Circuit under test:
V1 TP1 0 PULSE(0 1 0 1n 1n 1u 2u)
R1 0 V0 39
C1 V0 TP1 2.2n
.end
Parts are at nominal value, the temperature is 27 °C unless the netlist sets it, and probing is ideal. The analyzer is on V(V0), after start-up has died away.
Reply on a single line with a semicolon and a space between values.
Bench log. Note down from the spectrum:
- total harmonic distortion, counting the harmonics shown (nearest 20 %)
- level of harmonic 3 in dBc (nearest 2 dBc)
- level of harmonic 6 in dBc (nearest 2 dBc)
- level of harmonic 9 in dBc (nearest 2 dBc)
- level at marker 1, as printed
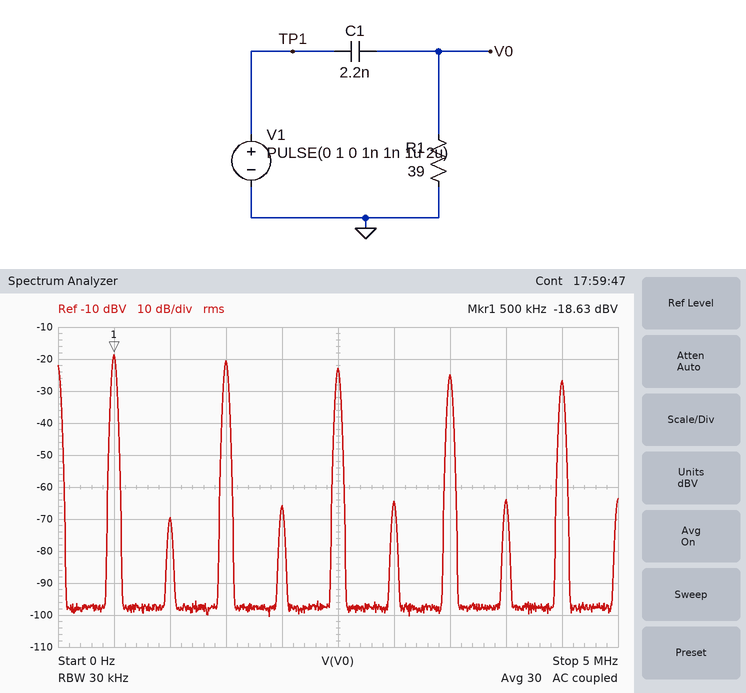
120 %; -2 dBc; -46 dBc; -8 dBc; -18.63 dBV
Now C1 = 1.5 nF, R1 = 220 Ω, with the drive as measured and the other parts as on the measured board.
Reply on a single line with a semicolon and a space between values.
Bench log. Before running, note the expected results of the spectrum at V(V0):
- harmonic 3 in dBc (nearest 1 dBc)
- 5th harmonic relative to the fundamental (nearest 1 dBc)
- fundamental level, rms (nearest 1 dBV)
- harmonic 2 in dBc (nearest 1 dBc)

-7 dBc; -11 dBc; -10 dBV; -54 dBc
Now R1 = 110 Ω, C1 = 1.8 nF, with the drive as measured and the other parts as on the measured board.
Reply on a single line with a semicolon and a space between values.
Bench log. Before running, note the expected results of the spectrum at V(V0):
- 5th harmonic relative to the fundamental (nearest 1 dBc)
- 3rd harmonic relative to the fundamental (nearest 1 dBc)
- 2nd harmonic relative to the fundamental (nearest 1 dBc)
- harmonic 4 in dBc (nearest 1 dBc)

-9 dBc; -5 dBc; -53 dBc; -51 dBc
